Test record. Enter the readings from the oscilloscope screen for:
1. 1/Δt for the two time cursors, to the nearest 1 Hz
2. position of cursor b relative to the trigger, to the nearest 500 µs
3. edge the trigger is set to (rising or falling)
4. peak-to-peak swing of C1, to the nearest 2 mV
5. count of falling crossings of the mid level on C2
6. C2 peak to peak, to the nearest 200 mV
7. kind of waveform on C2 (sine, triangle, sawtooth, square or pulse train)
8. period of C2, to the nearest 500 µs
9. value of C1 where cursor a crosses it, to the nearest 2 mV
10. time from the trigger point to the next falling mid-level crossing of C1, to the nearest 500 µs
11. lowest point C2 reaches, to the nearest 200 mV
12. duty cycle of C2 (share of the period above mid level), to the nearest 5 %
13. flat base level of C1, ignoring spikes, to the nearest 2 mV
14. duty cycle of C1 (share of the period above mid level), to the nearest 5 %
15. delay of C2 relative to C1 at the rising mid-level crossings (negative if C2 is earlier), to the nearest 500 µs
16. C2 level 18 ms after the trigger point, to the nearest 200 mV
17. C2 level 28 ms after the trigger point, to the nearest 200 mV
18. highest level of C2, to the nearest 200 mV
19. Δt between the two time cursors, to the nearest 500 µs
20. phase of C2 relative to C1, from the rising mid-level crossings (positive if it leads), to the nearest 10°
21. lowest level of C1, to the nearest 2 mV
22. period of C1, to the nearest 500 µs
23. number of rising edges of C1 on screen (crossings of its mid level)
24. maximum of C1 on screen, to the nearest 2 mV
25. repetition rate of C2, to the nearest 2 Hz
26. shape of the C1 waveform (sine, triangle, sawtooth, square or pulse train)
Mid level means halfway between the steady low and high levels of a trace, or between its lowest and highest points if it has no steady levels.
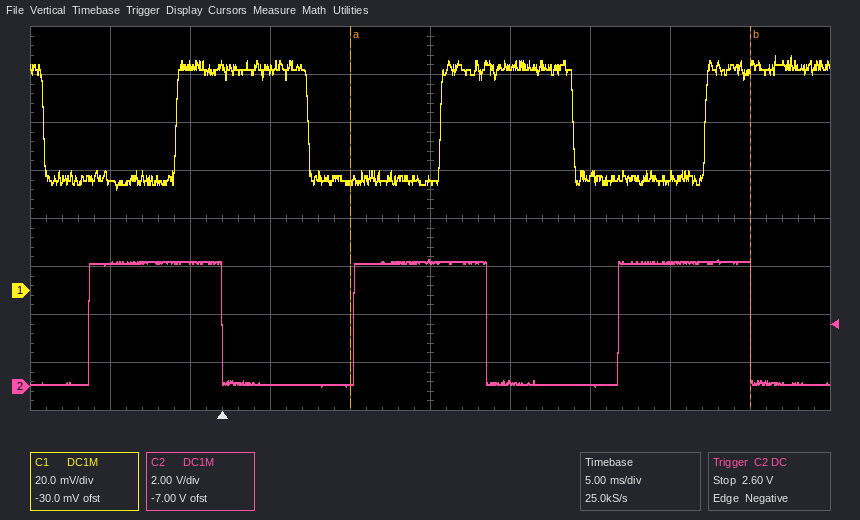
40 Hz
+33.0 ms
falling
56 mV
3
5.2 V
square
16.5 ms
46 mV
5.5 ms
0.0 V
50 %
46 mV
50 %
-5.5 ms
200 mV
5.2 V
5.2 V
25.0 ms
+120°
42 mV
16.5 ms
3
98 mV
60 Hz
square
